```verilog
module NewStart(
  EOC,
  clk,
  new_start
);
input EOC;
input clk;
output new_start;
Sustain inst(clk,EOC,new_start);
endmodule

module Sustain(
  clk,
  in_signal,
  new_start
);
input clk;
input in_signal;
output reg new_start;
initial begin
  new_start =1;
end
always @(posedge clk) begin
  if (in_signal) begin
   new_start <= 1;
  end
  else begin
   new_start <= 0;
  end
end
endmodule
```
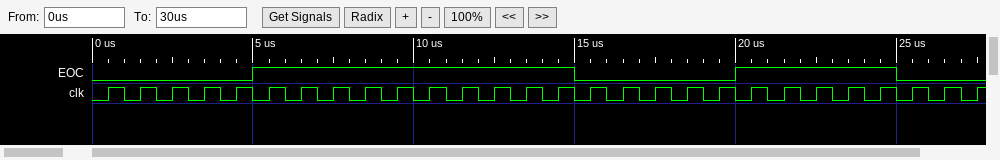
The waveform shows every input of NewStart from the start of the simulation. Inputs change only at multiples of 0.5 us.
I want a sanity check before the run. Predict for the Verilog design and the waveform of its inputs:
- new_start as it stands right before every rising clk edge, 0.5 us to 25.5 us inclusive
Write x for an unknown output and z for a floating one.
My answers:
1 0 0 0 0 0 1 1 1 1 1 1 1 1 1 1 0 0 0 0 0 1 1 1 1 1
